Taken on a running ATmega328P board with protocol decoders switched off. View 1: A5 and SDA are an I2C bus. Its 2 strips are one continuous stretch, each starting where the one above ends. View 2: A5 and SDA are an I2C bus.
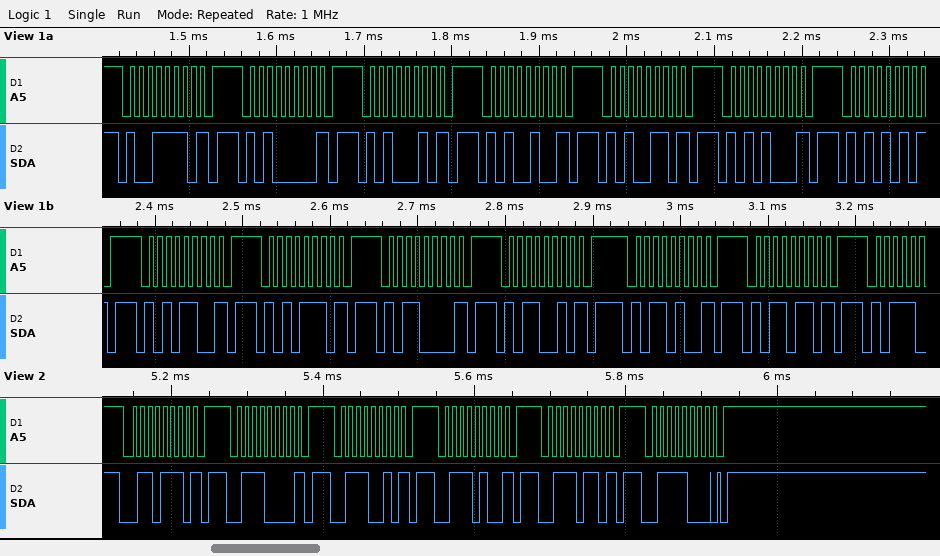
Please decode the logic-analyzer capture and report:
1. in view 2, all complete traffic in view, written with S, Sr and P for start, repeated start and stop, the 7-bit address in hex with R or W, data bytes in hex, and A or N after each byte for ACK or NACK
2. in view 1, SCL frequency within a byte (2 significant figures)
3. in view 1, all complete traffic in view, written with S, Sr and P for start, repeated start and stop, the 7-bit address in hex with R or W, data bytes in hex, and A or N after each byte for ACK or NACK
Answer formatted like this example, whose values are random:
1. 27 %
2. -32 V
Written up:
1. S 37W N P S 38W N P S 39W N P S 3AW N P S 3BW N P S 3CW A P
2. 100 kHz
3. S 4FW N P S 50W N P S 51W N P S 52W N P S 53W N P S 54W N P S 55W N P S 56W N P S 57W N P S 58W N P S 59W N P S 5AW N P S 5BW N P
